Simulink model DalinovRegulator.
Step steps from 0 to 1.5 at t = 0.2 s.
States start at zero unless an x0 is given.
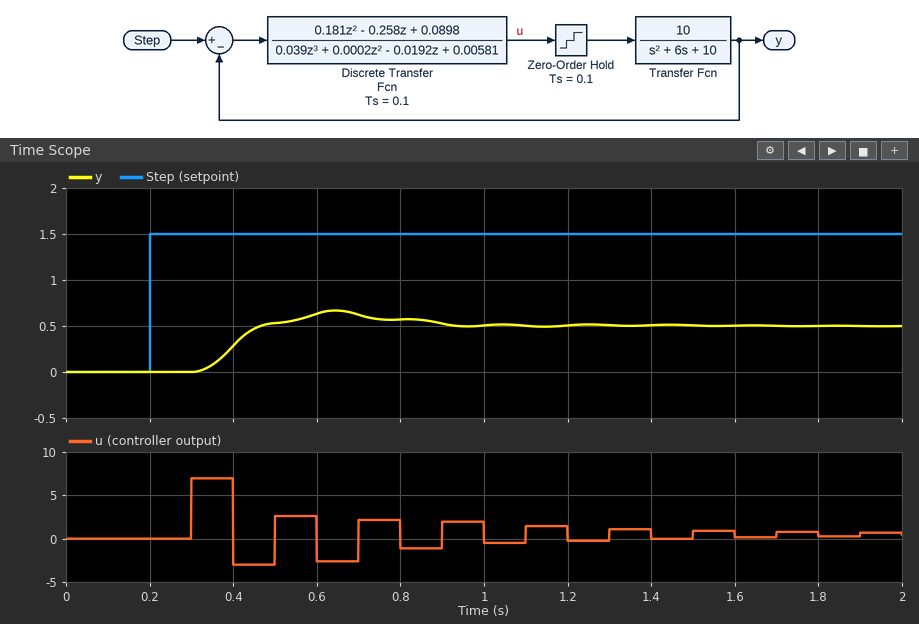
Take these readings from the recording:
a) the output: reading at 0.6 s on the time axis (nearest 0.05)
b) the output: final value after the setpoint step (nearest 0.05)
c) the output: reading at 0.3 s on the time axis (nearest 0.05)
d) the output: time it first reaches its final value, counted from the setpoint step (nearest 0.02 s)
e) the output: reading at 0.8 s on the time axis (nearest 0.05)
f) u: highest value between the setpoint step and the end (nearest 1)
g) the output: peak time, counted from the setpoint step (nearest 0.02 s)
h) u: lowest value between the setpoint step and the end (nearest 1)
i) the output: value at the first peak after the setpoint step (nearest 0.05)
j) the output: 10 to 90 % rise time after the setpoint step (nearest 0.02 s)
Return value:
0.65
0.50
0.00
0.26 s
0.55
7
0.44 s
-3
0.65
0.10 s
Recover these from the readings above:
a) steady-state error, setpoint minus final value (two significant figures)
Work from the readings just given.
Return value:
1.0
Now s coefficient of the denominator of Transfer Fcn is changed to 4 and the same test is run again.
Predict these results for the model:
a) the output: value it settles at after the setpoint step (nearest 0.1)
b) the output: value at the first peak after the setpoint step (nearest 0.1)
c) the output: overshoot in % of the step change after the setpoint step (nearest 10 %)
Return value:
0.5
0.8
70 %
